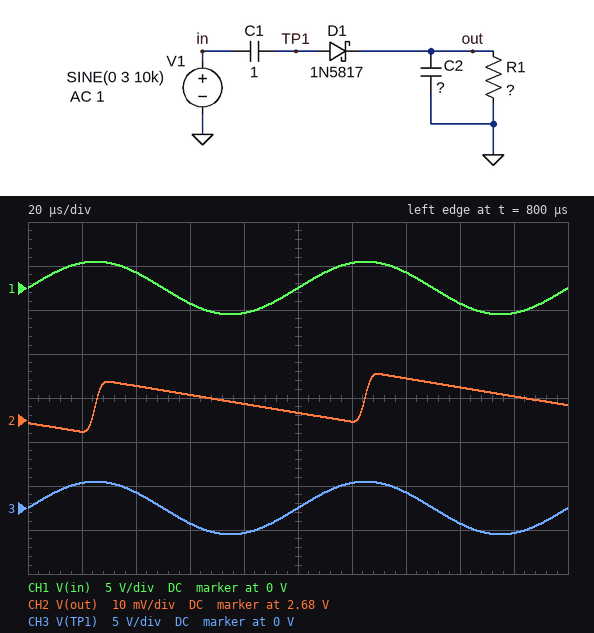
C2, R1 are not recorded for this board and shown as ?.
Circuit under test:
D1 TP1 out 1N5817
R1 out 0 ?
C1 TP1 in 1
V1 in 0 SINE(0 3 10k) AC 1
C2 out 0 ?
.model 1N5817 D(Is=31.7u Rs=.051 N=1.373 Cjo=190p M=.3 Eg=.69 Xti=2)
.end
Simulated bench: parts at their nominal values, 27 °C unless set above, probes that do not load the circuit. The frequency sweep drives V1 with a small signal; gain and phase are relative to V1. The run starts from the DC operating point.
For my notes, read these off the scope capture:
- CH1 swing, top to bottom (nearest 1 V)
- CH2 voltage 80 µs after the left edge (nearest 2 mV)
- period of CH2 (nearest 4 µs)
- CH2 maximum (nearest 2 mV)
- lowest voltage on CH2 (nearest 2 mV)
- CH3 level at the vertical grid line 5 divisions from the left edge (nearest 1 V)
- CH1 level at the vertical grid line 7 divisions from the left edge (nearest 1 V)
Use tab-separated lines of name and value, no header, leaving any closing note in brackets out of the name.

CH1 swing, top to bottom	6 V
CH2 voltage 80 µs after the left edge	2.684 V
period of CH2	100 µs
CH2 maximum	2.690 V
lowest voltage on CH2	2.678 V
CH3 level at the vertical grid line 5 divisions from the left edge	0 V
CH1 level at the vertical grid line 7 divisions from the left edge	2 V
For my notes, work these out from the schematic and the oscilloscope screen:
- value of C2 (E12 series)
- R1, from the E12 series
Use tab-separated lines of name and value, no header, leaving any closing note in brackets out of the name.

value of C2	68 µF
R1, from the E12 series	390 Ω
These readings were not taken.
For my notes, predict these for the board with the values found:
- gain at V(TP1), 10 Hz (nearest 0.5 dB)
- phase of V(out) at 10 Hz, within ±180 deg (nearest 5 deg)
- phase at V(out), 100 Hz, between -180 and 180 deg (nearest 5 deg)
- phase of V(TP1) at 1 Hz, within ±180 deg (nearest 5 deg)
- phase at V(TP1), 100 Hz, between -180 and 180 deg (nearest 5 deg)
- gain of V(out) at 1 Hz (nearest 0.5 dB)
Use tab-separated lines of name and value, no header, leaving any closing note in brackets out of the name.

gain at V(TP1), 10 Hz	0 dB
phase of V(out) at 10 Hz, within ±180 deg	-50 deg
phase at V(out), 100 Hz, between -180 and 180 deg	-85 deg
phase of V(TP1) at 1 Hz, within ±180 deg	0 deg
phase at V(TP1), 100 Hz, between -180 and 180 deg	0 deg
gain of V(out) at 1 Hz	-12.0 dB
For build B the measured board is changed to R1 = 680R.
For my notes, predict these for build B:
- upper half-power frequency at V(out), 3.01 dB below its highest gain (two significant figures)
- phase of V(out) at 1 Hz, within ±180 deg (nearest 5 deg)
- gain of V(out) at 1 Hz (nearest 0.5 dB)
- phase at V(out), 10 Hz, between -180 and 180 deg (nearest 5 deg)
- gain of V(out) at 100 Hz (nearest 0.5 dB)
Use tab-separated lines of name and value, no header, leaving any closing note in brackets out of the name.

upper half-power frequency at V(out), 3.01 dB below its highest gain	5.5 Hz
phase of V(out) at 1 Hz, within ±180 deg	-10 deg
gain of V(out) at 1 Hz	-8.5 dB
phase at V(out), 10 Hz, between -180 and 180 deg	-60 deg
gain of V(out) at 100 Hz	-33.5 dB
